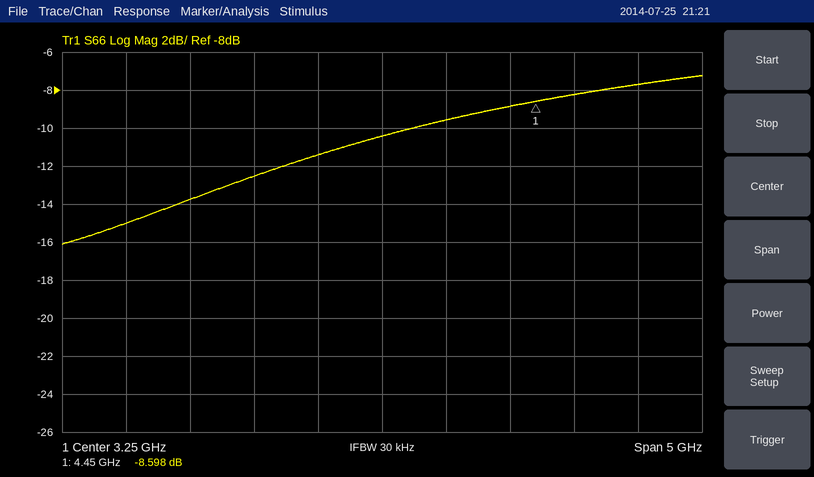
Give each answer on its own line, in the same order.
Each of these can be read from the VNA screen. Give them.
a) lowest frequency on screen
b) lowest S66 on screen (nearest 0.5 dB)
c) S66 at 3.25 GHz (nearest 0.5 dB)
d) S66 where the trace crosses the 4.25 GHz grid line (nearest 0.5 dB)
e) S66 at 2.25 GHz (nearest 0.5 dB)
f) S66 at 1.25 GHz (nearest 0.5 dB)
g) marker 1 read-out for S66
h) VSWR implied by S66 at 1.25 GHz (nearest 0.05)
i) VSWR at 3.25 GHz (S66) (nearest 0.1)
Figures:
750 MHz
-16.0 dB
-10.5 dB
-9.0 dB
-12.5 dB
-15.0 dB
-8.598 dB
1.45
1.9
